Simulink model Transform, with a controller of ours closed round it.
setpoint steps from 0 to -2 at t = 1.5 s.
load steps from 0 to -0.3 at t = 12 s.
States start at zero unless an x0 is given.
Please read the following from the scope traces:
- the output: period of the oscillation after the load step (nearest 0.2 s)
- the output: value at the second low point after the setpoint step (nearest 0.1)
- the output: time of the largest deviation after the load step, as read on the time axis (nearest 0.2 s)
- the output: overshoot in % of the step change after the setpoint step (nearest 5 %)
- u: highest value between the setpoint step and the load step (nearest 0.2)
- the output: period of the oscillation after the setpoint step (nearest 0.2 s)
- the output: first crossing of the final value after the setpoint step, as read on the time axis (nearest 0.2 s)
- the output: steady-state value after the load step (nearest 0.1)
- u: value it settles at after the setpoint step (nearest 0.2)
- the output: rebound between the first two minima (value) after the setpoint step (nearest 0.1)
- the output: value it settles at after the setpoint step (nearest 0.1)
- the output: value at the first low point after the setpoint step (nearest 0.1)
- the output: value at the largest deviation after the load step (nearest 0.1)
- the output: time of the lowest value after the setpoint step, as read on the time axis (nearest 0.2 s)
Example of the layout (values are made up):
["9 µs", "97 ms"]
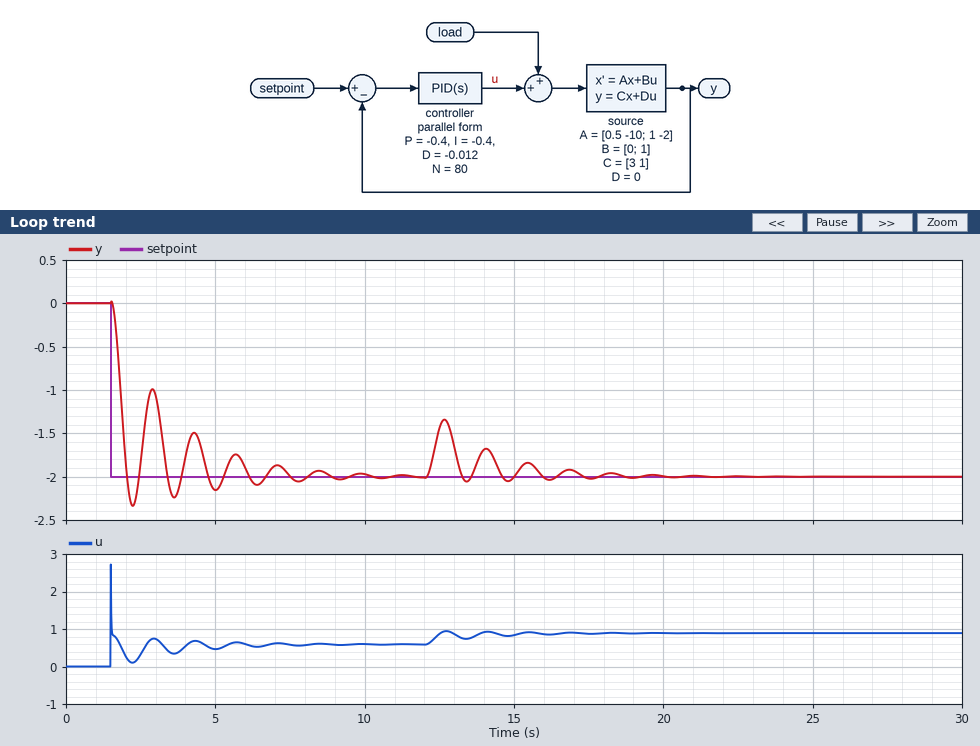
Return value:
["1.4 s", "-2.2", "12.6 s", "15 %", "2.8", "1.4 s", "2.0 s", "-2.0", "0.6", "-1.0", "-2.0", "-2.3", "-1.3", "2.2 s"]
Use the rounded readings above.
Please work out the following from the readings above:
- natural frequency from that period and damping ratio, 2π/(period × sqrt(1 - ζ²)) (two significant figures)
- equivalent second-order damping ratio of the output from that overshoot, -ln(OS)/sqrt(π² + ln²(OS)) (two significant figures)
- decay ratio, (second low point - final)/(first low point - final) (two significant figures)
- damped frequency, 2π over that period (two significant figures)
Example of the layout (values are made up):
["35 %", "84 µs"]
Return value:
["5.3 rad/s", "0.52", "0.67", "4.5 rad/s"]
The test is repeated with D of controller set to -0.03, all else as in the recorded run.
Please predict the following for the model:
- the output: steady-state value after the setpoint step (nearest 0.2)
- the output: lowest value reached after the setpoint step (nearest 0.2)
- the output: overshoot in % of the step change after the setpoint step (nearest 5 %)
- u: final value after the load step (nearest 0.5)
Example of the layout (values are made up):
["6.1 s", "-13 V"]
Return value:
["-2.0", "-2.2", "10 %", "1.0"]
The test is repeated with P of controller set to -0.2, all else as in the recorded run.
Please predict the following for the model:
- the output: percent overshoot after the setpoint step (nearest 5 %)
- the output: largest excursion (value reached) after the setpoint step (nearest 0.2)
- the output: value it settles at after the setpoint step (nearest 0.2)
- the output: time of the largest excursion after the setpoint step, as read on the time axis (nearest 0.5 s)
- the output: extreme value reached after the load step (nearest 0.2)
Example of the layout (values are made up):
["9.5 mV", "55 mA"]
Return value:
["10 %", "-2.2", "-2.0", "4.0 s", "-1.2"]
